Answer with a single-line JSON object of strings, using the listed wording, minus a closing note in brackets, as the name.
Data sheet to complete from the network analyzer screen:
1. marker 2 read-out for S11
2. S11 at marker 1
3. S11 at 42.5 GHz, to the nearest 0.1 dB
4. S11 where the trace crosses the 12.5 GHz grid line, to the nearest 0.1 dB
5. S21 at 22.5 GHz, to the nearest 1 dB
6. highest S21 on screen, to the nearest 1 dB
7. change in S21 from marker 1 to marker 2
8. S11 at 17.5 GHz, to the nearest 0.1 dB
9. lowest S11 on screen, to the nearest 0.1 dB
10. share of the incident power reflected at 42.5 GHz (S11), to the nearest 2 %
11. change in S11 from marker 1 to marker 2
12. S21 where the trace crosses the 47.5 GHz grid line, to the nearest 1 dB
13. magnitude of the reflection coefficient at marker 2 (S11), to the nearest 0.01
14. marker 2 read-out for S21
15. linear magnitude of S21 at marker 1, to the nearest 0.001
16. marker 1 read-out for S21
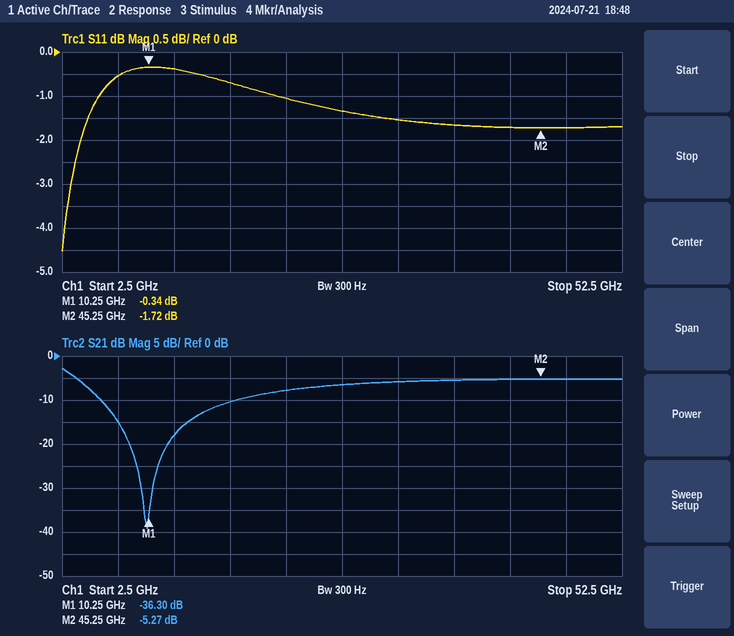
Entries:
{"marker 2 read-out for S11": "-1.72 dB", "S11 at marker 1": "-0.34 dB", "S11 at 42.5 GHz, to the nearest 0.1 dB": "-1.7 dB", "S11 where the trace crosses the 12.5 GHz grid line, to the nearest 0.1 dB": "-0.4 dB", "S21 at 22.5 GHz, to the nearest 1 dB": "-8 dB", "highest S21 on screen, to the nearest 1 dB": "-3 dB", "change in S21 from marker 1 to marker 2": "31.03 dB", "S11 at 17.5 GHz, to the nearest 0.1 dB": "-0.7 dB", "lowest S11 on screen, to the nearest 0.1 dB": "-4.5 dB", "share of the incident power reflected at 42.5 GHz (S11), to the nearest 2 %": "68 %", "change in S11 from marker 1 to marker 2": "-1.38 dB", "S21 where the trace crosses the 47.5 GHz grid line, to the nearest 1 dB": "-5 dB", "magnitude of the reflection coefficient at marker 2 (S11), to the nearest 0.01": "0.82", "marker 2 read-out for S21": "-5.27 dB", "linear magnitude of S21 at marker 1, to the nearest 0.001": "0.015", "marker 1 read-out for S21": "-36.30 dB"}
